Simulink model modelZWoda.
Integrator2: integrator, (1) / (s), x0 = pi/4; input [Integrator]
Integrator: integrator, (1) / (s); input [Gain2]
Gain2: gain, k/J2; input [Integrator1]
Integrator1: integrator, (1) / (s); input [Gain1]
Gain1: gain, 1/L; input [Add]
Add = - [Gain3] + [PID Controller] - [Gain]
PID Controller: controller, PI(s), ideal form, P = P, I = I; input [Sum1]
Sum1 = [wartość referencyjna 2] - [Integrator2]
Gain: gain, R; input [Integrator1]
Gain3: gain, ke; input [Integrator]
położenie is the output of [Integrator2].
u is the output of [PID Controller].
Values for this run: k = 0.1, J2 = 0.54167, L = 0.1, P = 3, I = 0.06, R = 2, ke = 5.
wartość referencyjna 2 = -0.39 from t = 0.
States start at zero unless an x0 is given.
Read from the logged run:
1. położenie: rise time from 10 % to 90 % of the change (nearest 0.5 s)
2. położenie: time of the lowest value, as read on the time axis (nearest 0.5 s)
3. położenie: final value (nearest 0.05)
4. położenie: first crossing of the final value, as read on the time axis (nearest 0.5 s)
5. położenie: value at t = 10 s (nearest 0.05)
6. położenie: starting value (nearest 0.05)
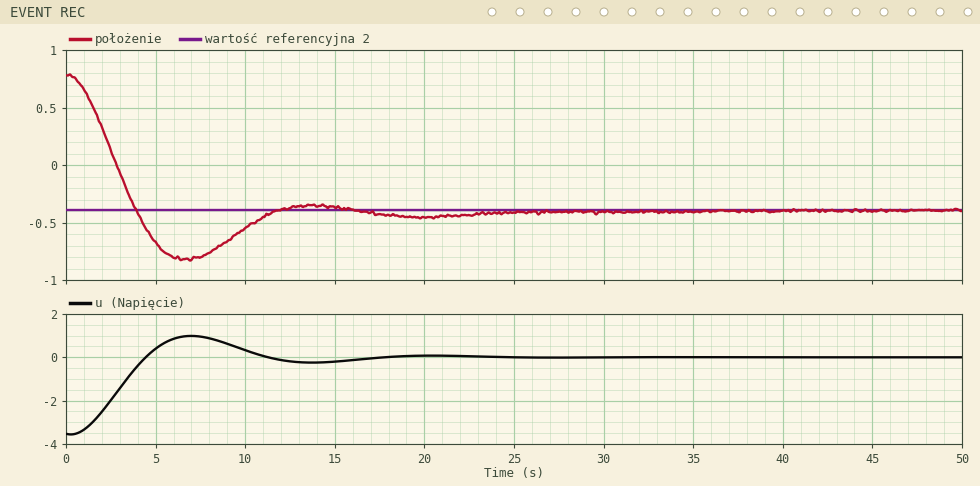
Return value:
2.5 s
6.5 s
-0.40
4.0 s
-0.55
0.80
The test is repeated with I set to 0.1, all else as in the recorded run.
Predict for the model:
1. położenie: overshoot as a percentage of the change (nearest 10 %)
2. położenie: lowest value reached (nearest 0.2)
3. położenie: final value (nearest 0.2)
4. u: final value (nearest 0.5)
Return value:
50 %
-1.0
-0.4
0.0
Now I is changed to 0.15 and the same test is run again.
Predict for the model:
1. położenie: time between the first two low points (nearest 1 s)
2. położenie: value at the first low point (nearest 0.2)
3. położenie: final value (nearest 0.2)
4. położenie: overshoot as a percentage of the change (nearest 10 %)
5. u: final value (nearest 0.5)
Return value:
14 s
-1.0
-0.4
60 %
0.0
